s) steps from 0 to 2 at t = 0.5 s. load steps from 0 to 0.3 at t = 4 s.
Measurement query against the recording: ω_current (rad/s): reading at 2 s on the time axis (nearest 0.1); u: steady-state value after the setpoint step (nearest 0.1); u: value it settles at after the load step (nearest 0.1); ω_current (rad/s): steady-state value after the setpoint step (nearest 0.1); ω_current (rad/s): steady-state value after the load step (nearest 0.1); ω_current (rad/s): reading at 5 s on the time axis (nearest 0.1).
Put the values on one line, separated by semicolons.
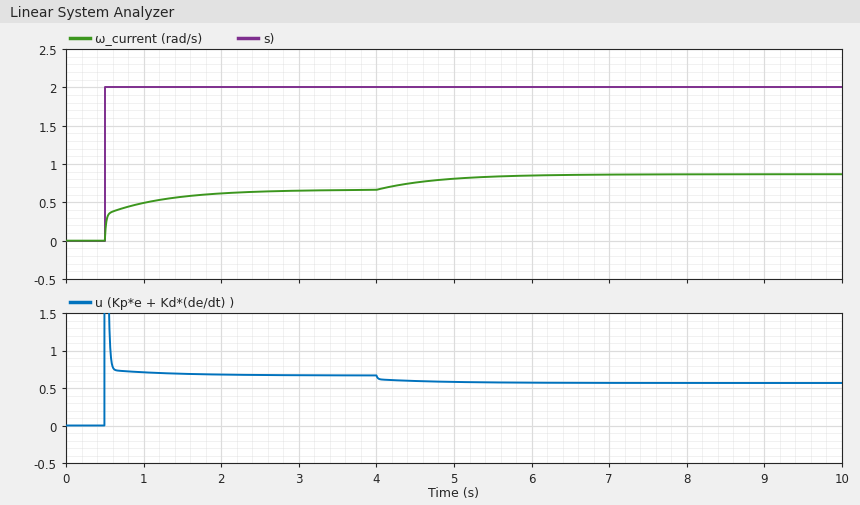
0.6; 0.7; 0.6; 0.7; 0.9; 0.8
